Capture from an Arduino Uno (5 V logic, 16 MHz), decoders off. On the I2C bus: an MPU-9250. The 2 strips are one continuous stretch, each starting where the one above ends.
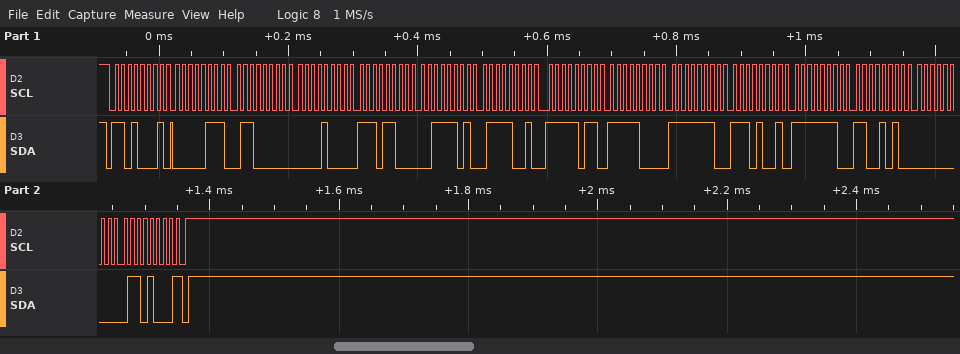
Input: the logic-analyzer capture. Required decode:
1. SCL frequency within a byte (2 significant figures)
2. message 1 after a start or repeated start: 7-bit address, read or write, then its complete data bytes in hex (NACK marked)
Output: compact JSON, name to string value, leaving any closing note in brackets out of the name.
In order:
{"SCL frequency within a byte": "100 kHz", "message 1 after a start or repeated start: 7-bit address, read or write, then its complete data bytes in hex": "0x68 read: 07 60 08 EC 3D 79 FB F8 FE E9 FE CA 00 68 NACK"}
